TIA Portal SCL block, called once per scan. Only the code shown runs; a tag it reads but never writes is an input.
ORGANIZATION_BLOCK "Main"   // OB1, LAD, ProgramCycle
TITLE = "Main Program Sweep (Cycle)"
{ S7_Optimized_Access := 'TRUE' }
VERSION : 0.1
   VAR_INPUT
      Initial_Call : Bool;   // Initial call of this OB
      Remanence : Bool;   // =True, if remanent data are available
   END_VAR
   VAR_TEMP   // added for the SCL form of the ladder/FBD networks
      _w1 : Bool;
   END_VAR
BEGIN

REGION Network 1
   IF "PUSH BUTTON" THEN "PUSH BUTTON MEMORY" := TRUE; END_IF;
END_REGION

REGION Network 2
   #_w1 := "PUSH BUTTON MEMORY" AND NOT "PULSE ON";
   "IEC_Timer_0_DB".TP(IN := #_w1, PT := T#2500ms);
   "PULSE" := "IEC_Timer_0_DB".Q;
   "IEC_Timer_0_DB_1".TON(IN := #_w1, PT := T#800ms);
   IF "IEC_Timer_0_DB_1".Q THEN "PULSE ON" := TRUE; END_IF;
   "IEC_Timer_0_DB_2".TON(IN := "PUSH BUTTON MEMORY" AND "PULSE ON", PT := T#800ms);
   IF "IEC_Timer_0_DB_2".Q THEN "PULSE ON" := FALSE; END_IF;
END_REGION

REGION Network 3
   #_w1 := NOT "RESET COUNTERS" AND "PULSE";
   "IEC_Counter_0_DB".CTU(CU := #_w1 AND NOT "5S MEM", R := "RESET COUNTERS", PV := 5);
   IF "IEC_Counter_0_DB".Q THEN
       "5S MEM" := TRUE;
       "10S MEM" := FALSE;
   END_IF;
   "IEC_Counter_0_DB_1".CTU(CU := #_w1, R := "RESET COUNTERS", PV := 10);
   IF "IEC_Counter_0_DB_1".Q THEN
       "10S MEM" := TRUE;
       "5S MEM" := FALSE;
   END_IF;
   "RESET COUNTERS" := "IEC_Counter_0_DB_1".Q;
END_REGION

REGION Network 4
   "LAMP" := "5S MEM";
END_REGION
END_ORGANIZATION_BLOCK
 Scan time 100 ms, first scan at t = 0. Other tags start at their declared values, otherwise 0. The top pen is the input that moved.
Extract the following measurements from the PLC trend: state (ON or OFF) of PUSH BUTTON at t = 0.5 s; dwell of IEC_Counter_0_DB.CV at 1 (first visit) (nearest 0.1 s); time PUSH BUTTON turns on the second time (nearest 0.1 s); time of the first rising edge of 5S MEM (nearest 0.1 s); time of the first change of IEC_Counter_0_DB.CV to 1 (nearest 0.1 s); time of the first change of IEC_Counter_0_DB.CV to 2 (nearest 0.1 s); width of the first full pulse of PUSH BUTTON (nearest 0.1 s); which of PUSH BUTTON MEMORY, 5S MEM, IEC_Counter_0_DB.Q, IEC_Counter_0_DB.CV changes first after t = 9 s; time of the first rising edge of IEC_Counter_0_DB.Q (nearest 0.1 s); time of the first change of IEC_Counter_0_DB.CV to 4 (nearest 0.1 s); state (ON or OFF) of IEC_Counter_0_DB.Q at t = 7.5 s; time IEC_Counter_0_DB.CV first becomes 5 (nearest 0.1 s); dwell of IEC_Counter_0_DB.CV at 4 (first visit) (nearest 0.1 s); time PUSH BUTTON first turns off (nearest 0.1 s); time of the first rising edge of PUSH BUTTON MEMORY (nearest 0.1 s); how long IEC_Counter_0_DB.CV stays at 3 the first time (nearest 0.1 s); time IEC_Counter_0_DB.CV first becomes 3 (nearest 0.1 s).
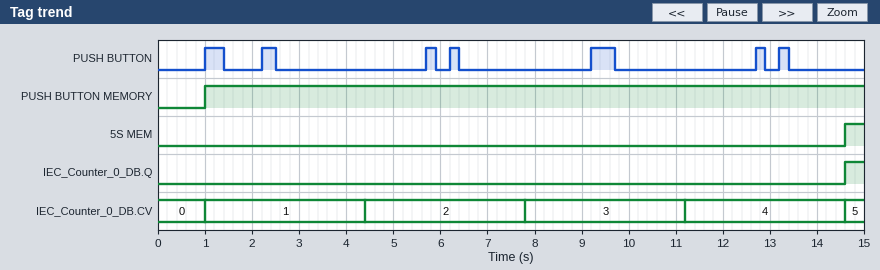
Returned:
OFF
3.4 s
2.2 s
14.6 s
1.0 s
4.4 s
0.4 s
IEC_Counter_0_DB.CV
14.6 s
11.2 s
OFF
14.6 s
3.4 s
1.4 s
1.0 s
3.4 s
7.8 s
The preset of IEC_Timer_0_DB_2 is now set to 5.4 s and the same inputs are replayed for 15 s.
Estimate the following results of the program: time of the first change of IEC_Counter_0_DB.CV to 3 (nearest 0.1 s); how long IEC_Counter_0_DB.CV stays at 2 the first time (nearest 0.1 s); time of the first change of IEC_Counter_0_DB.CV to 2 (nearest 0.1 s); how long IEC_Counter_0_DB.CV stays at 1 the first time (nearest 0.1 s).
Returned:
13.6 s
6.3 s
7.3 s
6.3 s
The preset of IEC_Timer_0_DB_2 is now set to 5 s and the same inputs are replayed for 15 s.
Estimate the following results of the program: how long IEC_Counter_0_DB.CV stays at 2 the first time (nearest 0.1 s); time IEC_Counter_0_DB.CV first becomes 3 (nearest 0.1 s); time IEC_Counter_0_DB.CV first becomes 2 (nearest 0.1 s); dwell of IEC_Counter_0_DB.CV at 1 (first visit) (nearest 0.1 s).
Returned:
5.9 s
12.8 s
6.9 s
5.9 s
